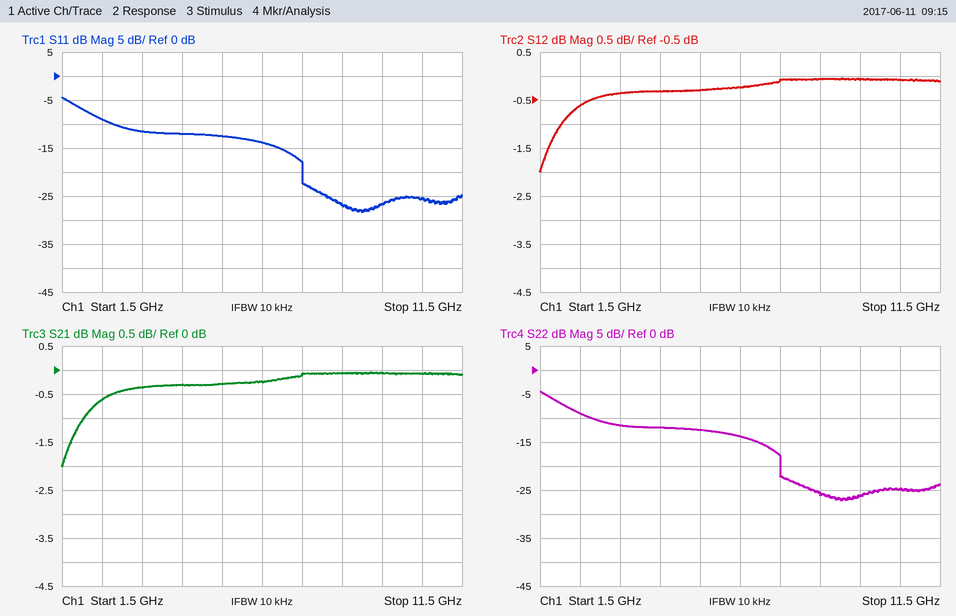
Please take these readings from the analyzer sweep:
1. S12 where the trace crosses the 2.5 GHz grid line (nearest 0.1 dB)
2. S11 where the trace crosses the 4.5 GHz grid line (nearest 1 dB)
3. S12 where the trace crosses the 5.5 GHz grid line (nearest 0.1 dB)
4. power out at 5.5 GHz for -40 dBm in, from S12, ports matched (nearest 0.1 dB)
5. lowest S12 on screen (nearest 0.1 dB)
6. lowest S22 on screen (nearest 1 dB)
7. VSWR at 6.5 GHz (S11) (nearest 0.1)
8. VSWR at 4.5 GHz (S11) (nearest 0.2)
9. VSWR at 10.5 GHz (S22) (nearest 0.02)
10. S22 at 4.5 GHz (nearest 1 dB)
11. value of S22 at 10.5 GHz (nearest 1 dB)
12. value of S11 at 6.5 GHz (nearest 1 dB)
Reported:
-0.6 dB
-12 dB
-0.3 dB
-40.3 dBm
-2.0 dB
-27 dB
1.5
1.6
1.12
-12 dB
-25 dB
-14 dB
